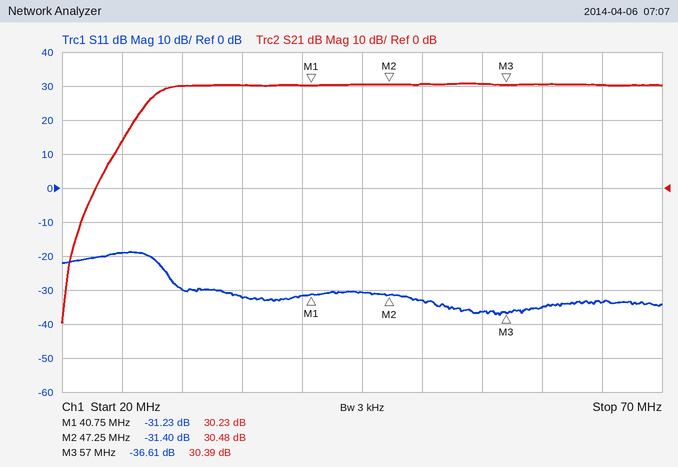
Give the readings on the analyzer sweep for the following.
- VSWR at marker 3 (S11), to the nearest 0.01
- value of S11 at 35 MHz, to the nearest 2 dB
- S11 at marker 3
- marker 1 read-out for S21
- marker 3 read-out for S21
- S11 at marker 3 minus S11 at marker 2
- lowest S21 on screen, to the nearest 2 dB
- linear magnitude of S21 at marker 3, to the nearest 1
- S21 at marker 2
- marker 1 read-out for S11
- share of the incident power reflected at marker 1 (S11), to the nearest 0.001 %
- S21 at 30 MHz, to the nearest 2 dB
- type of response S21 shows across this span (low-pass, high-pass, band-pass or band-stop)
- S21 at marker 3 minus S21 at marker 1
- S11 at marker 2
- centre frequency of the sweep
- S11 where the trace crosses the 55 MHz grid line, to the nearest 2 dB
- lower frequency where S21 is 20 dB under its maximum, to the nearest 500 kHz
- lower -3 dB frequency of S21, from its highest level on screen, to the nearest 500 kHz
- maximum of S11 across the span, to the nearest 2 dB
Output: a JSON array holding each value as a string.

["1.03", "-32 dB", "-36.61 dB", "30.23 dB", "30.39 dB", "-5.21 dB", "-40 dB", "33", "30.48 dB", "-31.23 dB", "0.075 %", "30 dB", "high-pass", "0.16 dB", "-31.40 dB", "45 MHz", "-36 dB", "24.5 MHz", "28.0 MHz", "-18 dB"]
